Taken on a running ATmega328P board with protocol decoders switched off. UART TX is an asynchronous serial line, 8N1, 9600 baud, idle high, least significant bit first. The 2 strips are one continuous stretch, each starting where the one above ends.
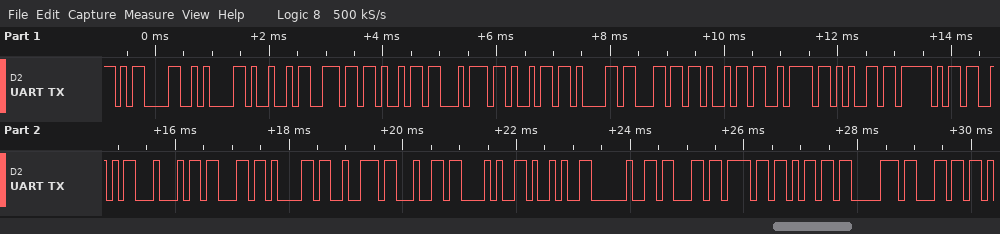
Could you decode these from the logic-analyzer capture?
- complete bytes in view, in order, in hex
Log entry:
0D 0A 49 6E 69 74 69 61 6C 69 7A 65 5F 53 44 63 61 72 64 28 29 20 63 6F 6D 70 6C
